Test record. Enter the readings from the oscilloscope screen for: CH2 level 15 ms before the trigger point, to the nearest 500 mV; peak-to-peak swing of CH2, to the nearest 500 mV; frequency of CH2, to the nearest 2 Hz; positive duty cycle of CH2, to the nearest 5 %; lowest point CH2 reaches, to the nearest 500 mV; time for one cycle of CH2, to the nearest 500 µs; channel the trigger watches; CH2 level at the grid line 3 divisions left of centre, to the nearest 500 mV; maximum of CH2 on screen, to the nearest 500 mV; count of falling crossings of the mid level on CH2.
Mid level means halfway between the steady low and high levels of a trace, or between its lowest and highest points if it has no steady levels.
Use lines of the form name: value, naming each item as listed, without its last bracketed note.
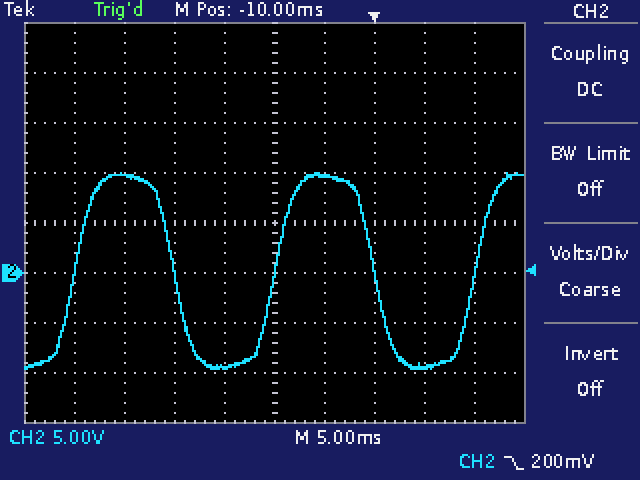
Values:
CH2 level 15 ms before the trigger point, to the nearest 500 mV: -9.5 V
peak-to-peak swing of CH2, to the nearest 500 mV: 19.5 V
frequency of CH2, to the nearest 2 Hz: 50 Hz
positive duty cycle of CH2, to the nearest 5 %: 50 %
lowest point CH2 reaches, to the nearest 500 mV: -9.5 V
time for one cycle of CH2, to the nearest 500 µs: 20.0 ms
channel the trigger watches: CH2
CH2 level at the grid line 3 divisions left of centre, to the nearest 500 mV: 10.0 V
maximum of CH2 on screen, to the nearest 500 mV: 10.0 V
count of falling crossings of the mid level on CH2: 2
